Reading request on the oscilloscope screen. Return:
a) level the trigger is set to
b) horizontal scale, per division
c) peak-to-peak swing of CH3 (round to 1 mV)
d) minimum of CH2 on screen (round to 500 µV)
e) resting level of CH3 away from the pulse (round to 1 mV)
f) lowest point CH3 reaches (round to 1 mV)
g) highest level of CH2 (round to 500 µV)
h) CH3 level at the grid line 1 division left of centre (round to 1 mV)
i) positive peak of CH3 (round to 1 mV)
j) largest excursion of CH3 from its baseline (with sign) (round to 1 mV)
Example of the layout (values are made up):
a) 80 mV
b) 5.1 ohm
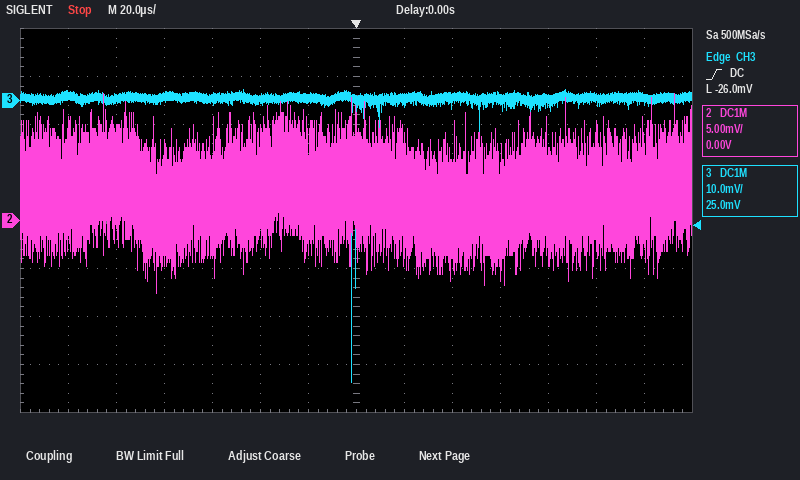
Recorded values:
a) -26.0 mV
b) 20 µs
c) 61 mV
d) -7.5 mV
e) 0 mV
f) -59 mV
g) 13.0 mV
h) 0 mV
i) 2 mV
j) -59 mV
